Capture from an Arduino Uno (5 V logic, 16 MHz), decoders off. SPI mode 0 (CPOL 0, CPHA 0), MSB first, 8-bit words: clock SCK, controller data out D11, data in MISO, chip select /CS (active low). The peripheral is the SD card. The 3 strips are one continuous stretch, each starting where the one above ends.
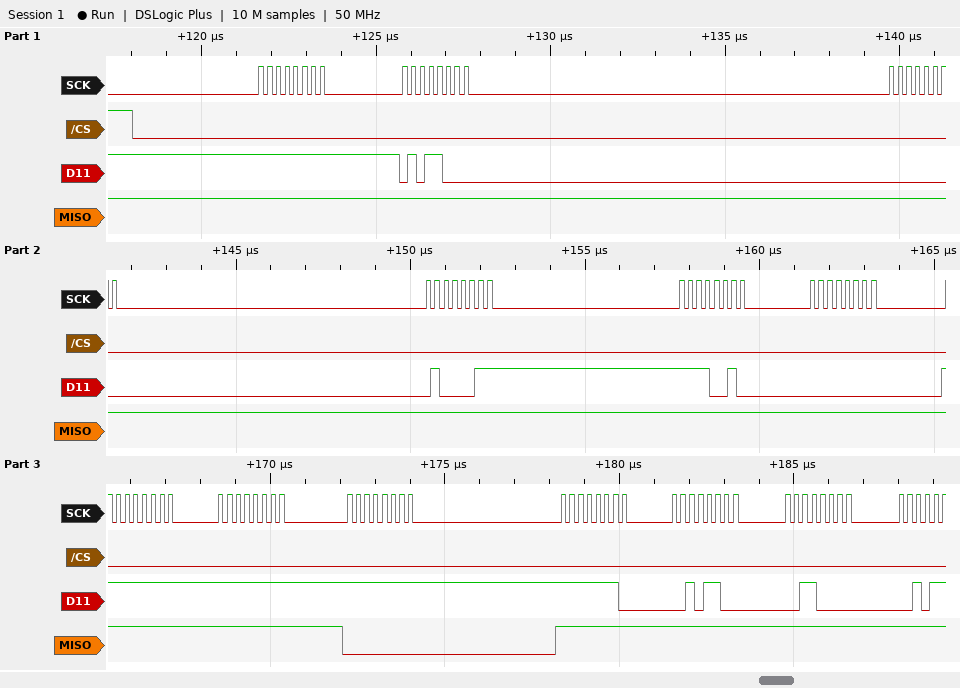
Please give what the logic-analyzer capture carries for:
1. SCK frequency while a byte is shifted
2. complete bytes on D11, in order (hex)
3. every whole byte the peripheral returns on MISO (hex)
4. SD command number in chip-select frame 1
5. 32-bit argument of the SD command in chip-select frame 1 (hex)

4 MHz
0xFF 0x58 0x00 0x43 0xF2 0x00 0xFF 0xFF 0xFF 0xFE 0x2C 0x30
0xFF 0xFF 0xFF 0xFF 0xFF 0xFF 0xFF 0xFF 0x00 0xFF 0xFF 0xFF
CMD24
0x0043F200
